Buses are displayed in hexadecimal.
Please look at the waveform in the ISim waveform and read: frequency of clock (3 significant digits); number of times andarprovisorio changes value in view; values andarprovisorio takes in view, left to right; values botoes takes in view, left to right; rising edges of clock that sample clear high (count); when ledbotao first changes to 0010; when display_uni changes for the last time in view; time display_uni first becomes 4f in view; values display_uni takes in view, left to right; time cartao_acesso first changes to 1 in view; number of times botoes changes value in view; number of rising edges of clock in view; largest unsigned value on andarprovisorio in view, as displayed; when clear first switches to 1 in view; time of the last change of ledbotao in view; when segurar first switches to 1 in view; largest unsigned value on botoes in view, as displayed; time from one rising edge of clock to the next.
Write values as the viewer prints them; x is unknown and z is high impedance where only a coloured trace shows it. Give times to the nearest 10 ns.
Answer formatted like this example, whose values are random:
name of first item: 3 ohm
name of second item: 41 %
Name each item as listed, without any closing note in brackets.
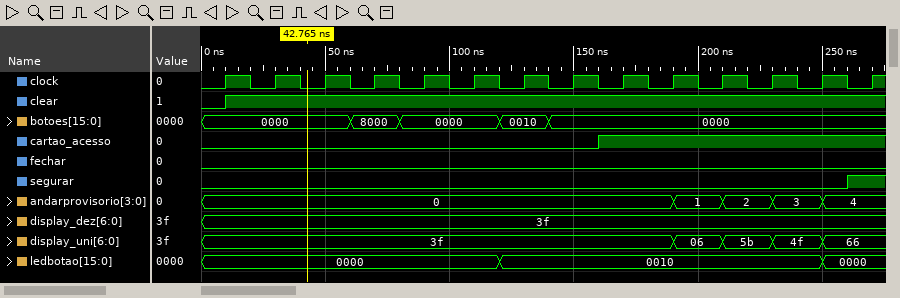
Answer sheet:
frequency of clock: 50.0 MHz
number of times andarprovisorio changes value in view: 4
values andarprovisorio takes in view, left to right: 0, 1, 2, 3, 4
values botoes takes in view, left to right: 0000, 8000, 0000, 0010, 0000
rising edges of clock that sample clear high: 13
when ledbotao first changes to 0010: 120 ns
when display_uni changes for the last time in view: 250 ns
time display_uni first becomes 4f in view: 230 ns
values display_uni takes in view, left to right: 3f, 06, 5b, 4f, 66
time cartao_acesso first changes to 1 in view: 160 ns
number of times botoes changes value in view: 4
number of rising edges of clock in view: 14
largest unsigned value on andarprovisorio in view, as displayed: 4
when clear first switches to 1 in view: 10 ns
time of the last change of ledbotao in view: 250 ns
when segurar first switches to 1 in view: 260 ns
largest unsigned value on botoes in view, as displayed: 8000
time from one rising edge of clock to the next: 20 ns
